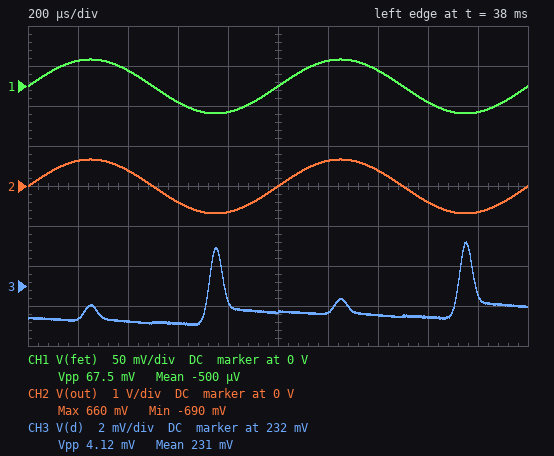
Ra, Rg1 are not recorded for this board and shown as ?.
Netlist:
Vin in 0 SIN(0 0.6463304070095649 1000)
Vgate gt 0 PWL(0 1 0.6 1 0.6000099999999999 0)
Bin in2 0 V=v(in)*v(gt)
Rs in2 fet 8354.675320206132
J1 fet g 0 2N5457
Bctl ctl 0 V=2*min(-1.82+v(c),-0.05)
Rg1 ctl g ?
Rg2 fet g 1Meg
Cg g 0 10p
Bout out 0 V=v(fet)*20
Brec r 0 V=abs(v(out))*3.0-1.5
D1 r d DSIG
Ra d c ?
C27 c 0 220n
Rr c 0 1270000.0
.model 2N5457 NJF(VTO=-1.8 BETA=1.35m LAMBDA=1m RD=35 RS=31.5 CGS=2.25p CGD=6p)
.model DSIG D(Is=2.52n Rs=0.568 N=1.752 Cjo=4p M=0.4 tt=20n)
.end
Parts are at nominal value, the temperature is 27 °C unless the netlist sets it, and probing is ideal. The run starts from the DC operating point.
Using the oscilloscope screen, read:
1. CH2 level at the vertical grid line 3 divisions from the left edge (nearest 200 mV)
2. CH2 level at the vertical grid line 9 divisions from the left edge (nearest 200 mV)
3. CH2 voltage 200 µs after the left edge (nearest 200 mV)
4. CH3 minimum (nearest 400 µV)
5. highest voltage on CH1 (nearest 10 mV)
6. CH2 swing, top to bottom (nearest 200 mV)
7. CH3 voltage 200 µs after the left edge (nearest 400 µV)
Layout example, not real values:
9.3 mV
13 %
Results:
-400 mV
-600 mV
600 mV
230.0 mV
30 mV
1.4 V
230.4 mV
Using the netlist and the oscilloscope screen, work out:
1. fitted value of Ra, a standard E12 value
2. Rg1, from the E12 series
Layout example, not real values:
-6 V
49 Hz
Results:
1 kΩ
2.7 MΩ
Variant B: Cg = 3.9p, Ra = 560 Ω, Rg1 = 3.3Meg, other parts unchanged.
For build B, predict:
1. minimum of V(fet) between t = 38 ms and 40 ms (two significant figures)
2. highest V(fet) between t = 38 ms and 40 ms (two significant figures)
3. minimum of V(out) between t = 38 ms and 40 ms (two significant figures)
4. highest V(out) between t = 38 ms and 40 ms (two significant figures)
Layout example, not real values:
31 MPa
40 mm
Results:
-32 mV
31 mV
-650 mV
630 mV
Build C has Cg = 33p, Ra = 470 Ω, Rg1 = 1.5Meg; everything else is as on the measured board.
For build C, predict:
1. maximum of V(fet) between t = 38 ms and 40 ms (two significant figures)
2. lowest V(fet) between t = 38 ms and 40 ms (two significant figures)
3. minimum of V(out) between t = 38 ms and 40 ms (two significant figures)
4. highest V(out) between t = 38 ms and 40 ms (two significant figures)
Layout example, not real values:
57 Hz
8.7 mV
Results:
39 mV
-40 mV
-800 mV
770 mV
